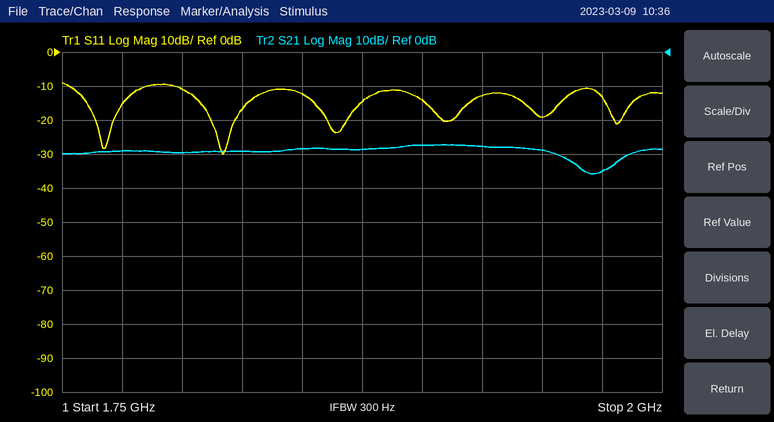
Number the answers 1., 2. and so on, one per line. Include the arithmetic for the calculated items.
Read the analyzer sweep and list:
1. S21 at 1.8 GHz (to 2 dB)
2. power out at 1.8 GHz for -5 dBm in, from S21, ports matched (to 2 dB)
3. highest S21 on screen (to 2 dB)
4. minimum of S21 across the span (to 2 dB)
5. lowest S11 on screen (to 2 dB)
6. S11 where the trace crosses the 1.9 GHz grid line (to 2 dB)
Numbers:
1. -30 dB
2. -5 dBm + (-30 dB) = -34 dBm
3. -28 dB
4. -36 dB
5. -30 dB
6. -14 dB
